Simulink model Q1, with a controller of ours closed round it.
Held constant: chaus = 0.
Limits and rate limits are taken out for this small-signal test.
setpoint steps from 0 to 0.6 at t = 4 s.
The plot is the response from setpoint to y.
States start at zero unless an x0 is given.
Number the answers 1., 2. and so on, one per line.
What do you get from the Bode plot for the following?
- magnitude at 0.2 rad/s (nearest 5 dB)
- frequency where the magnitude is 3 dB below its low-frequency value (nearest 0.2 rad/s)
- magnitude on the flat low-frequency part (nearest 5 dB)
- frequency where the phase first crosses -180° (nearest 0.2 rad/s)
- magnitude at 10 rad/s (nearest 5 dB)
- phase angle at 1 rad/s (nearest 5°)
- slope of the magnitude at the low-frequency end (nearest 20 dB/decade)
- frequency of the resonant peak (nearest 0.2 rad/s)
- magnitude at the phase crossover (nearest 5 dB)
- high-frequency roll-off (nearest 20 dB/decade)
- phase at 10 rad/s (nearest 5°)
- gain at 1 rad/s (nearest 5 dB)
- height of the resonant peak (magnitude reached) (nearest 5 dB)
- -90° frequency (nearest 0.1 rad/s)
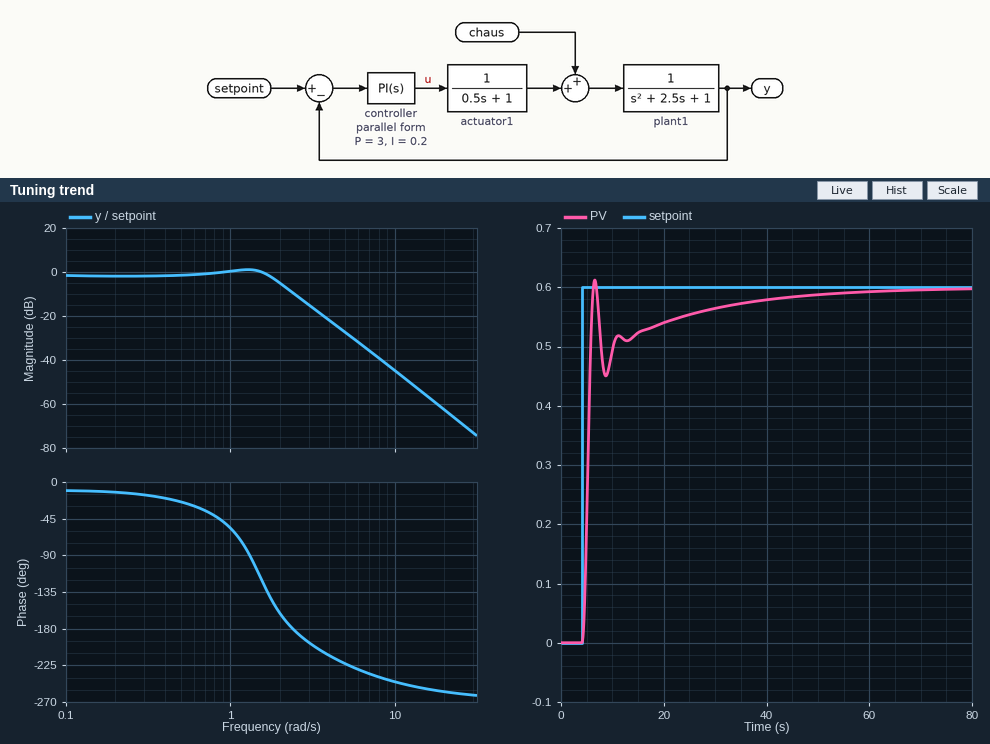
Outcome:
1. 0 dB
2. 2.0 rad/s
3. 0 dB
4. 2.4 rad/s
5. -45 dB
6. -55°
7. 0 dB/decade
8. 1.2 rad/s
9. -10 dB
10. -60 dB/decade
11. -245°
12. 0 dB
13. 0 dB
14. 1.3 rad/s
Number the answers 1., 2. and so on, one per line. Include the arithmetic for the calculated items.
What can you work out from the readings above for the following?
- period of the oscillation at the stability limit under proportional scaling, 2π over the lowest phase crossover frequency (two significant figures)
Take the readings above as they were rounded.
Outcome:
1. 2π / 2.4 = 2.6 s
